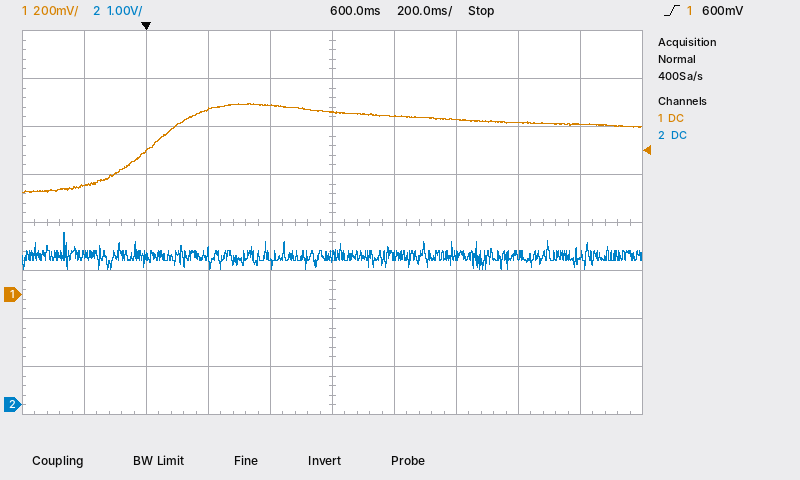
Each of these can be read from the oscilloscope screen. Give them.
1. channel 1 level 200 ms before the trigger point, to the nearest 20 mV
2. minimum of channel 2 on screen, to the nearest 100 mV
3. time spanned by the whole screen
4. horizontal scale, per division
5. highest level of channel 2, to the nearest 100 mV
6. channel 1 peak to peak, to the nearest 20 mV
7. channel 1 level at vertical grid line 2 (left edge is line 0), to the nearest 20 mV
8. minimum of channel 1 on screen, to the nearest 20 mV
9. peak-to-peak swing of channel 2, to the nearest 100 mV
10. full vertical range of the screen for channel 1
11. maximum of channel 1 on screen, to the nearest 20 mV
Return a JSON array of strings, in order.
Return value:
["460 mV", "2.8 V", "2 s", "200 ms", "3.6 V", "380 mV", "600 mV", "420 mV", "800 mV", "1.6 V", "800 mV"]
